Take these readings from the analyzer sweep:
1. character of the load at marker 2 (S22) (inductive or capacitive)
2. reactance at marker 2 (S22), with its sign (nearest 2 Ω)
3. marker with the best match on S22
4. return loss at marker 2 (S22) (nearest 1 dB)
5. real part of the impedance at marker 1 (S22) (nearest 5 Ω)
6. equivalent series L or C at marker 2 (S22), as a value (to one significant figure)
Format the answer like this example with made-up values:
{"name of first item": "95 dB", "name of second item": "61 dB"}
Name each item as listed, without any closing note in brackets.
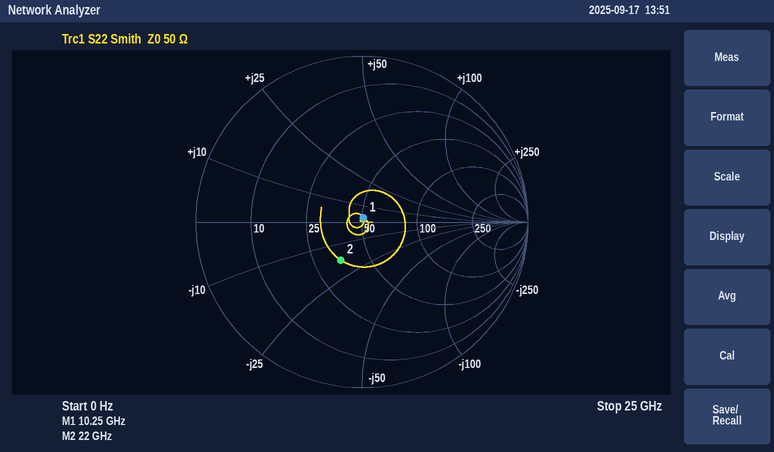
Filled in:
{"character of the load at marker 2 (S22)": "capacitive", "reactance at marker 2 (S22), with its sign": "-18 Ω", "marker with the best match on S22": "marker 1", "return loss at marker 2 (S22)": "12 dB", "real part of the impedance at marker 1 (S22)": "50 Ω", "equivalent series L or C at marker 2 (S22), as a value": "400 fF"}
